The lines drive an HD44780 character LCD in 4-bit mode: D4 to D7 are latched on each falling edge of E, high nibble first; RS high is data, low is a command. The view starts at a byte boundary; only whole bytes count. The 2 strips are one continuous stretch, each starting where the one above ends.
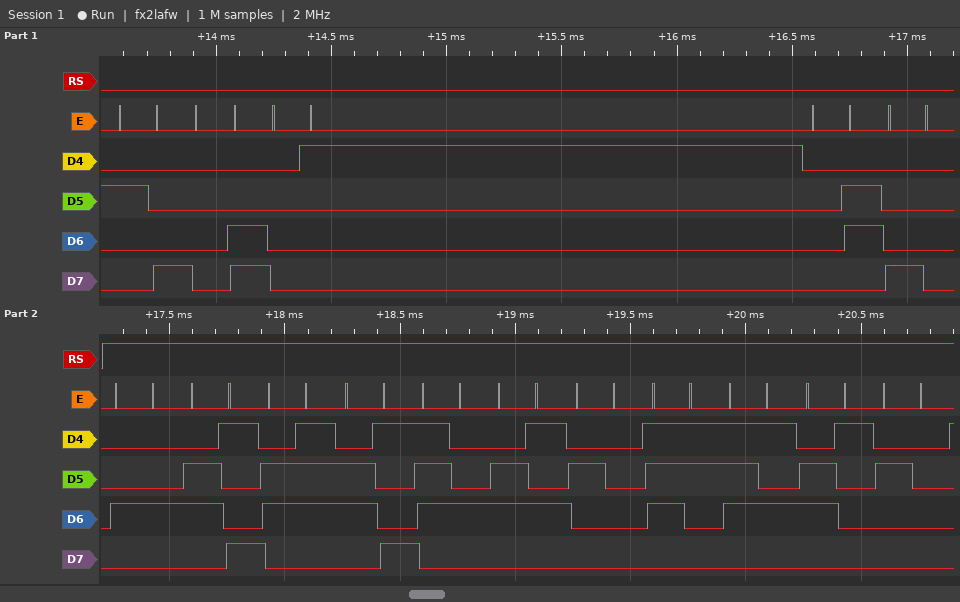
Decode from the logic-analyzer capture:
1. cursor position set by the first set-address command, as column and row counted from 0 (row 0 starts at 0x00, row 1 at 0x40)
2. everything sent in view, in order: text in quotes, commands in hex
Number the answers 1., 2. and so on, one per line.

1. column 0, row 0
2. 0x28 0x0C 0x01 0x06 0x80 "Digite sua "
